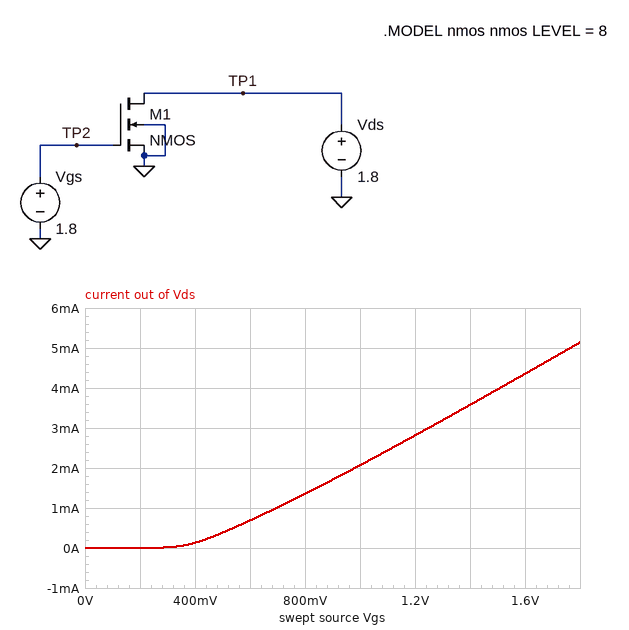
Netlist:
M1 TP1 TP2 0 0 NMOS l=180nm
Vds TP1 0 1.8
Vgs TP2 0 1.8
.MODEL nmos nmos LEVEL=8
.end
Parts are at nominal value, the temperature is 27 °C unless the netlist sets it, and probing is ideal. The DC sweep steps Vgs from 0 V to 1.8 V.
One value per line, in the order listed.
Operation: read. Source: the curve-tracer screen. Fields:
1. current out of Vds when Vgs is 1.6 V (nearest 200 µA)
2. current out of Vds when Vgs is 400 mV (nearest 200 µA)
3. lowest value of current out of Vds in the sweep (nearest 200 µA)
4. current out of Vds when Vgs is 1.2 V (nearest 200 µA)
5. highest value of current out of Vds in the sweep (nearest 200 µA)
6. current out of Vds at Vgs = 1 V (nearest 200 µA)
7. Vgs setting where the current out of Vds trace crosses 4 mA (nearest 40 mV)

4.4 mA
200 µA
0 A
2.8 mA
5.2 mA
2.0 mA
1.52 V
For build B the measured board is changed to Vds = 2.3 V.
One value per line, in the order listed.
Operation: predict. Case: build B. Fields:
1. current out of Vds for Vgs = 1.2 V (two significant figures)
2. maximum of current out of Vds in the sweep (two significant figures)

3.0 mA
5.4 mA
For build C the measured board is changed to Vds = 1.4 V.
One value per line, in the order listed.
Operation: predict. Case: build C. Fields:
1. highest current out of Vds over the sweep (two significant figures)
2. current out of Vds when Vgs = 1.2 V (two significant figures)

4.9 mA
2.7 mA
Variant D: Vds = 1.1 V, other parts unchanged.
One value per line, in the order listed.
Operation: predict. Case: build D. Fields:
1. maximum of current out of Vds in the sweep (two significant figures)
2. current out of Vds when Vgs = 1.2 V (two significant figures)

4.7 mA
2.6 mA
